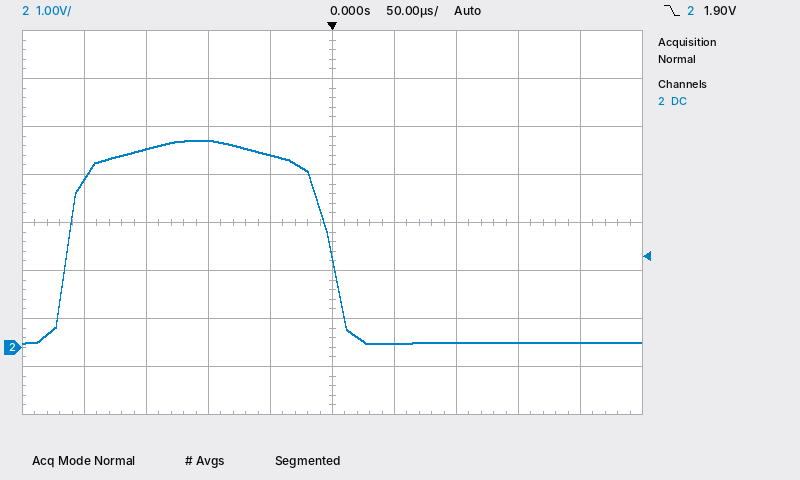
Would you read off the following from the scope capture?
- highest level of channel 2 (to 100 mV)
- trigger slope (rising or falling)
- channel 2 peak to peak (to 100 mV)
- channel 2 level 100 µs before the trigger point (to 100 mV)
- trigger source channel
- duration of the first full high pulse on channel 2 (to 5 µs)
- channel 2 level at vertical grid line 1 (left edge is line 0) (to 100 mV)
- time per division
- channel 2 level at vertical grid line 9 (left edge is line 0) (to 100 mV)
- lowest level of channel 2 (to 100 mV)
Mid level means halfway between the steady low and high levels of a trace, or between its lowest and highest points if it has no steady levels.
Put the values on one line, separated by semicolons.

4.3 V; falling; 4.2 V; 4.3 V; channel 2; 210 µs; 3.5 V; 50 µs; 100 mV; 100 mV
